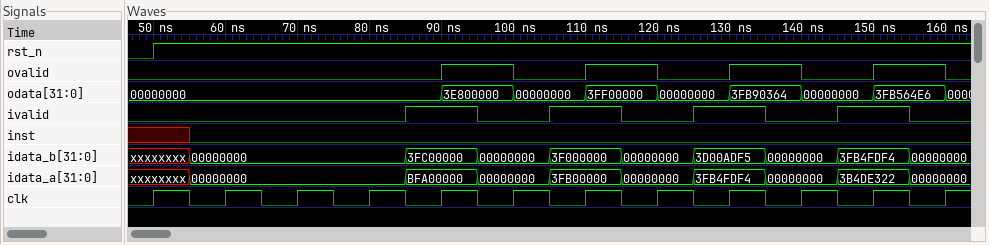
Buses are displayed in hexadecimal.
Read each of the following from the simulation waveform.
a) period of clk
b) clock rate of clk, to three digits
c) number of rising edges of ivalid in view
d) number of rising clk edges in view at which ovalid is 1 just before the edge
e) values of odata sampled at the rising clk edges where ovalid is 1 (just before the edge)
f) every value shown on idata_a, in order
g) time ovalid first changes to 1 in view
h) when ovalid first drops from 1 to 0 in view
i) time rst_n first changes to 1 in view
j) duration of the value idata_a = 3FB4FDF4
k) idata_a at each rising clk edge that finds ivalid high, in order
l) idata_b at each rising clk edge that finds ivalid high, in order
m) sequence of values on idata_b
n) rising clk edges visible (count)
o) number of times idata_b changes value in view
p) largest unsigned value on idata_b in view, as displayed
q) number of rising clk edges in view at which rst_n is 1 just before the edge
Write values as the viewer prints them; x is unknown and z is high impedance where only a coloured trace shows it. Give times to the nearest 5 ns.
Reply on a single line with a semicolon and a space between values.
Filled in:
10 ns; 100 MHz; 4; 4; 3E800000, 3FF00000, 3FB90364, 3FB564E6; xxxxxxxx, 00000000, BFA00000, 00000000, 3FB00000, 00000000, 3FB4FDF4, 00000000, 3B4DE322, 00000000; 90 ns; 100 ns; 50 ns; 10 ns; BFA00000, 3FB00000, 3FB4FDF4, 3B4DE322; 3FC00000, 3F000000, 3D00ADF5, 3FB4FDF4; xxxxxxxx, 00000000, 3FC00000, 00000000, 3F000000, 00000000, 3D00ADF5, 00000000, 3FB4FDF4, 00000000; 12; 9; 3FC00000; 11
